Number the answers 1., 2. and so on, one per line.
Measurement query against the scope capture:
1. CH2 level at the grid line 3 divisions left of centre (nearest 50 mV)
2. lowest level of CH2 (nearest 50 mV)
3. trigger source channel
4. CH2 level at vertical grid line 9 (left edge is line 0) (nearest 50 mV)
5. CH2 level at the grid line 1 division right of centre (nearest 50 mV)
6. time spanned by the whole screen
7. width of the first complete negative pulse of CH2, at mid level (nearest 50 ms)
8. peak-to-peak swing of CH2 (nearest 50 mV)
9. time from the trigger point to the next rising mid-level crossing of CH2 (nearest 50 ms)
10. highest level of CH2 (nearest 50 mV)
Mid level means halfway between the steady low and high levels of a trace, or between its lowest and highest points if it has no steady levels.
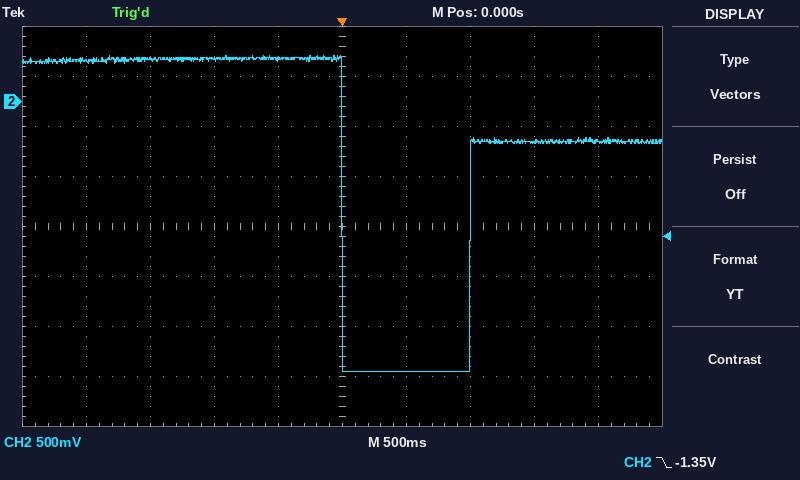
1. 400 mV
2. -2.70 V
3. CH2
4. -400 mV
5. -2.70 V
6. 5 s
7. 1.00 s
8. 3.15 V
9. 1.00 s
10. 450 mV
